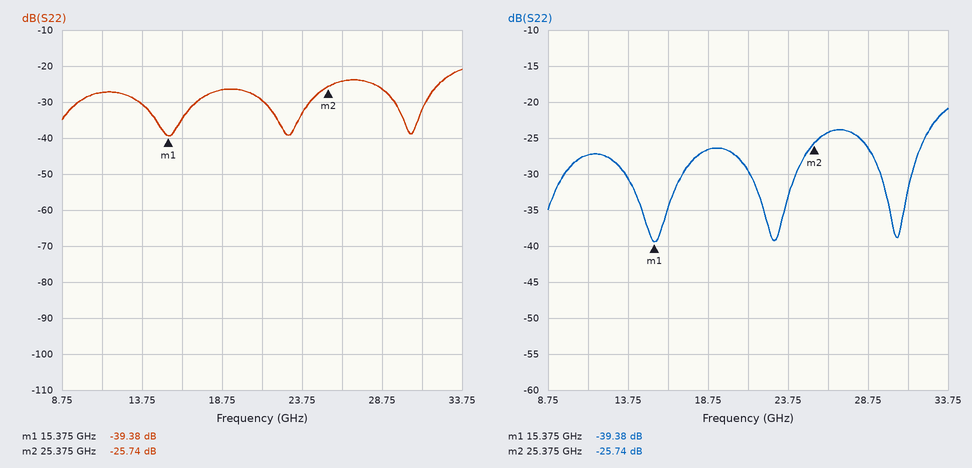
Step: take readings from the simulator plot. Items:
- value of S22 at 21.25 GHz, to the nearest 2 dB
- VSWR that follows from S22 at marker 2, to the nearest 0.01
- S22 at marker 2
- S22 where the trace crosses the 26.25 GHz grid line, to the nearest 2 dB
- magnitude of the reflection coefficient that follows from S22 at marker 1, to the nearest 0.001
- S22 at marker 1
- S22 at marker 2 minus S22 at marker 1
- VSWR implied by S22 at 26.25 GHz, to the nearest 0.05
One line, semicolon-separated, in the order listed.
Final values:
-30 dB; 1.11; -25.74 dB; -24 dB; 0.011; -39.38 dB; 13.64 dB; 1.15
